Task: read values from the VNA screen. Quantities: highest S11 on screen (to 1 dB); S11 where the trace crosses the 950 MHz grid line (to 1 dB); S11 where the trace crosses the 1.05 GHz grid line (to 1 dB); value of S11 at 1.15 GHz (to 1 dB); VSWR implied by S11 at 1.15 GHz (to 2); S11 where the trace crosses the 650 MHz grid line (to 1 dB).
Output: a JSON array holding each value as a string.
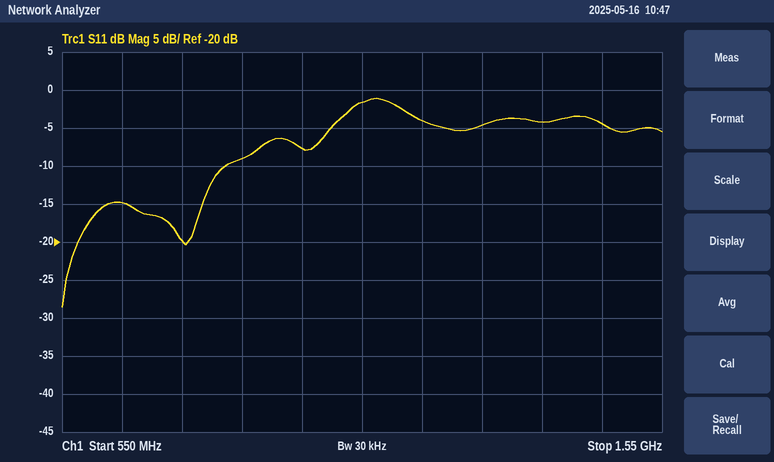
["-1 dB", "-8 dB", "-2 dB", "-4 dB", "4", "-15 dB"]
